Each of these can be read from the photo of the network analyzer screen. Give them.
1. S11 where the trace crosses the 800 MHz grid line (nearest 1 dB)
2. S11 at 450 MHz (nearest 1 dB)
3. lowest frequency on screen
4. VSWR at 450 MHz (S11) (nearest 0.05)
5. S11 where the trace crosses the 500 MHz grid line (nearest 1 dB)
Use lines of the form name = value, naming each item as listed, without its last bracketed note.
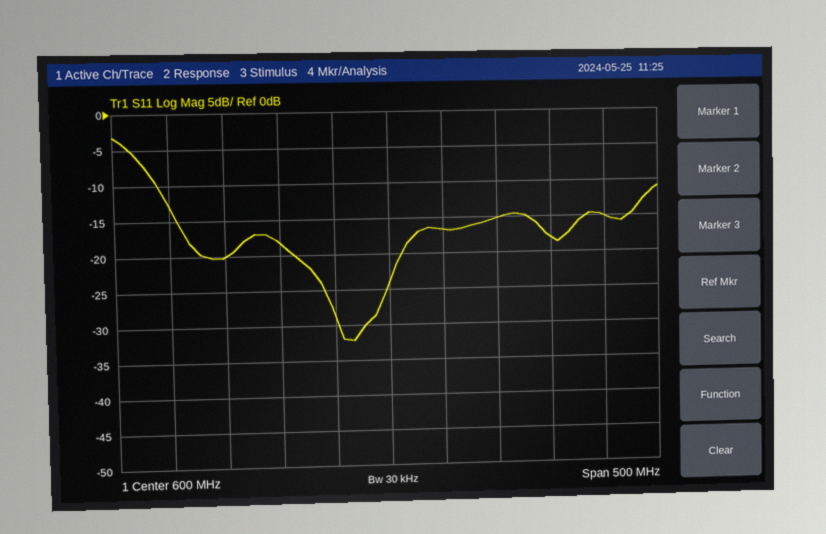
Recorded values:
S11 where the trace crosses the 800 MHz grid line = -15 dB
S11 at 450 MHz = -20 dB
lowest frequency on screen = 350 MHz
VSWR at 450 MHz (S11) = 1.20
S11 where the trace crosses the 500 MHz grid line = -18 dB
